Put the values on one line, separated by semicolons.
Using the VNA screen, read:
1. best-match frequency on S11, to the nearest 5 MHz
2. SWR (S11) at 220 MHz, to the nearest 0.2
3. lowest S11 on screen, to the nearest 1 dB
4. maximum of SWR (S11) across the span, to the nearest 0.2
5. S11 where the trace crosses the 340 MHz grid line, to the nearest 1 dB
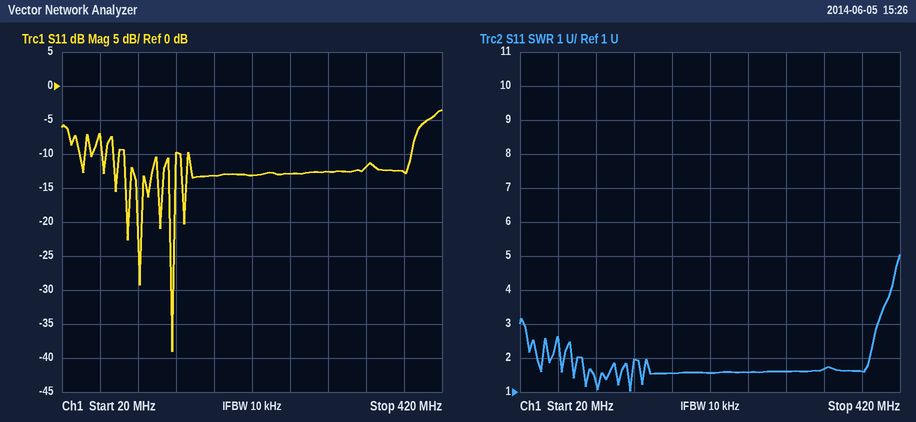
135 MHz; 1.6; -39 dB; 5.0; -12 dB
